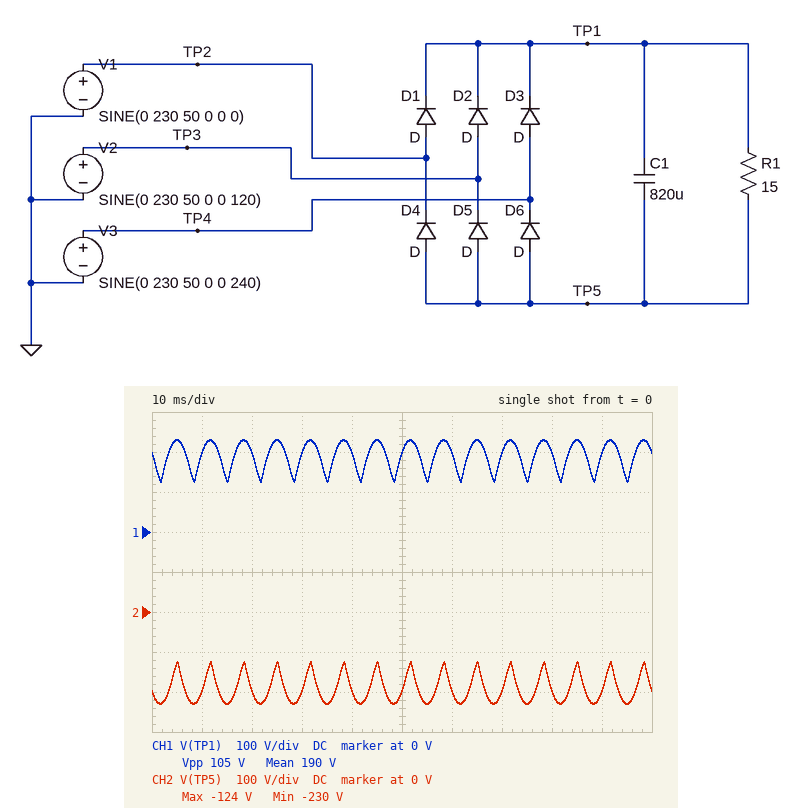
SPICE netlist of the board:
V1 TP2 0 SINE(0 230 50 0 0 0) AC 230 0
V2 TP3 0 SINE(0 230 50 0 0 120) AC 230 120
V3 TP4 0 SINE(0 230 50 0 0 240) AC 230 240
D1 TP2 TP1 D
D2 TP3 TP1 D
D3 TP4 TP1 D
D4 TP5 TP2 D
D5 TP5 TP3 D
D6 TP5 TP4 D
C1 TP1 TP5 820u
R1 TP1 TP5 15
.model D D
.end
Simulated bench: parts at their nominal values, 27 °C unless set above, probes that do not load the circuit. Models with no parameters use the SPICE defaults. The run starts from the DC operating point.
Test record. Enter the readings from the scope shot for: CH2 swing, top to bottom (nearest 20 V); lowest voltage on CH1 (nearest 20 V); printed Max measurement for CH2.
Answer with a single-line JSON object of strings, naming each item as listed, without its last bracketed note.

{"CH2 swing, top to bottom": "100 V", "lowest voltage on CH1": "120 V", "printed Max measurement for CH2": "-124 V"}
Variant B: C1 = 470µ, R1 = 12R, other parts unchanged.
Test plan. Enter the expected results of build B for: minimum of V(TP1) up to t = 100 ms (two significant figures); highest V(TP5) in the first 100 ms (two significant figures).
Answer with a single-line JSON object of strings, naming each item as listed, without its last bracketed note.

{"minimum of V(TP1) up to t = 100 ms": "110 V", "highest V(TP5) in the first 100 ms": "-110 V"}
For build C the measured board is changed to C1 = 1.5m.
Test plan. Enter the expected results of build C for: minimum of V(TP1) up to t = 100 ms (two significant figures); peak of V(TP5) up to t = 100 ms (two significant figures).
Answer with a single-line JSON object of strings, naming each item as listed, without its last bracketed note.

{"minimum of V(TP1) up to t = 100 ms": "140 V", "peak of V(TP5) up to t = 100 ms": "-140 V"}
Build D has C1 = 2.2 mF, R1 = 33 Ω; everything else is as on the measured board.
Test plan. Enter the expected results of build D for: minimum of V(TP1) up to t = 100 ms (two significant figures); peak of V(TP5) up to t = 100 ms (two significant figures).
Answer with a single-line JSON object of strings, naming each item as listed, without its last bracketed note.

{"minimum of V(TP1) up to t = 100 ms": "160 V", "peak of V(TP5) up to t = 100 ms": "-160 V"}
